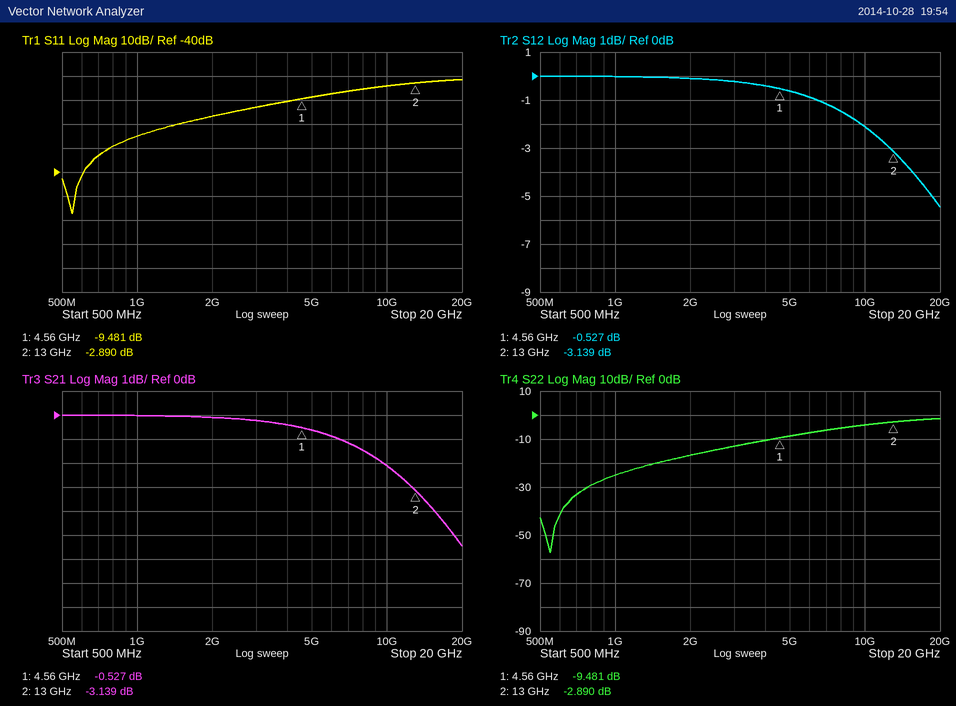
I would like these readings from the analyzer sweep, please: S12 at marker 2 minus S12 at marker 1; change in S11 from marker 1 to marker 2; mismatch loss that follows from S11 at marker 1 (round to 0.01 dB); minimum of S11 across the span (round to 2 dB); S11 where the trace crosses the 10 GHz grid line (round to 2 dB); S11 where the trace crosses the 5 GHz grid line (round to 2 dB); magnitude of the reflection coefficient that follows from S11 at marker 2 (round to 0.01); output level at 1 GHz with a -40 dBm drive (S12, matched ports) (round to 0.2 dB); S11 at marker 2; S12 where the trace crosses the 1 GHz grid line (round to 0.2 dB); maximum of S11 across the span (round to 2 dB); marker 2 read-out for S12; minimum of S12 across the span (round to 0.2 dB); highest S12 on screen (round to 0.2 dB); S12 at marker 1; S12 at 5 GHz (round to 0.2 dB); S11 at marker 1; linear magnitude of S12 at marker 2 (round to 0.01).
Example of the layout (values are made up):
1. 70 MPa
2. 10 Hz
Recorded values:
1. -2.612 dB
2. 6.591 dB
3. 0.52 dB
4. -58 dB
5. -4 dB
6. -8 dB
7. 0.72
8. -40.0 dBm
9. -2.890 dB
10. 0.0 dB
11. -2 dB
12. -3.139 dB
13. -5.4 dB
14. 0.0 dB
15. -0.527 dB
16. -0.6 dB
17. -9.481 dB
18. 0.70
